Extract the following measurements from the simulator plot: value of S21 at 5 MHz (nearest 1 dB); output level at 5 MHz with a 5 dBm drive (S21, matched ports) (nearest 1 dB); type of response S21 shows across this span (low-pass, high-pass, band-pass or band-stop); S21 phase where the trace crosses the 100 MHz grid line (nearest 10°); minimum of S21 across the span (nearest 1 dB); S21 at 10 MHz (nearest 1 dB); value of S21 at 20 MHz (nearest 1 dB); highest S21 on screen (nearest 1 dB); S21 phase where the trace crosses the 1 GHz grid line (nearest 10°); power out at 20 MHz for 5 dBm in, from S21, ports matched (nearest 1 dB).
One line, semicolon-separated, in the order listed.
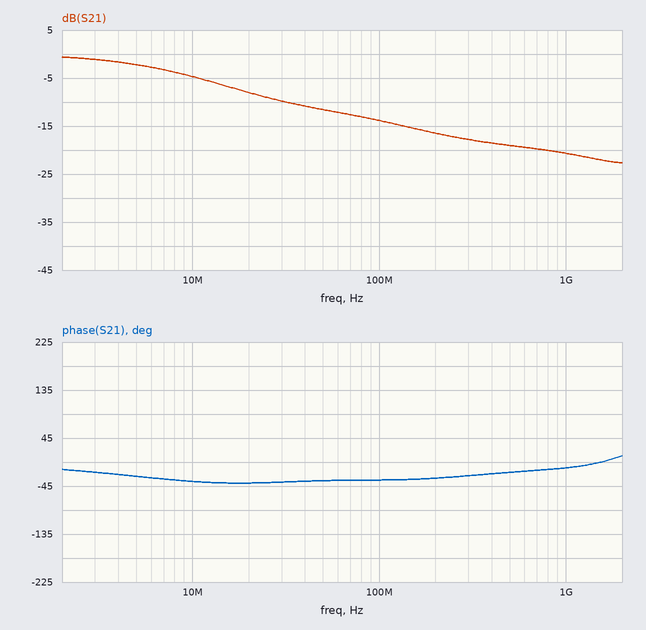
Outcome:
-2 dB; 3 dBm; low-pass; -30°; -23 dB; -5 dB; -8 dB; -1 dB; -10°; -3 dBm
